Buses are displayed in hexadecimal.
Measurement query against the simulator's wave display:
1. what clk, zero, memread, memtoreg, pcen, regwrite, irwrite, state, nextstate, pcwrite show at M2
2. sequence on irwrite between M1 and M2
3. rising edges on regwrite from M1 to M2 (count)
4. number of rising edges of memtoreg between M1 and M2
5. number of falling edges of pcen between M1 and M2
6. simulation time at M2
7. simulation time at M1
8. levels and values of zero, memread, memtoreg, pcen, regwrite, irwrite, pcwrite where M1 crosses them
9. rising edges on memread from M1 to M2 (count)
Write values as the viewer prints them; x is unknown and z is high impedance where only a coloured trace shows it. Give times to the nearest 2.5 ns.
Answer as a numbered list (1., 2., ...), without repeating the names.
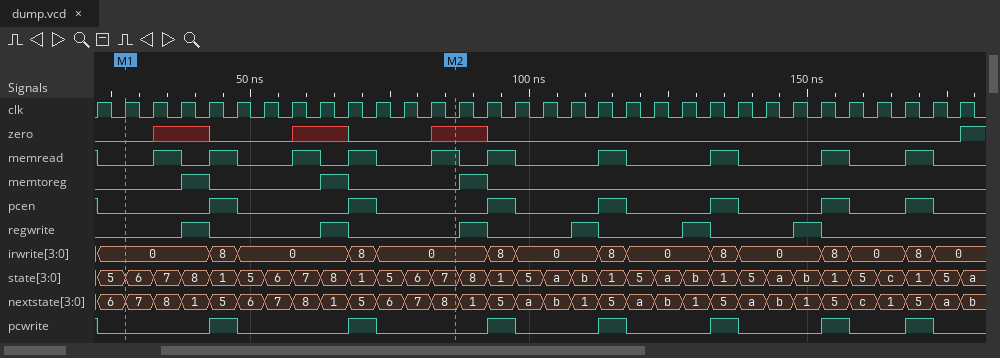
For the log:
1. clk=0, zero=x, memread=1, memtoreg=0, pcen=0, regwrite=0, irwrite=0, state=7, nextstate=8, pcwrite=0
2. 0, 8, 0, 8, 0
3. 2
4. 2
5. 2
6. 87.5 ns
7. 27.5 ns
8. zero=0, memread=0, memtoreg=0, pcen=0, regwrite=0, irwrite=0, pcwrite=0
9. 5
